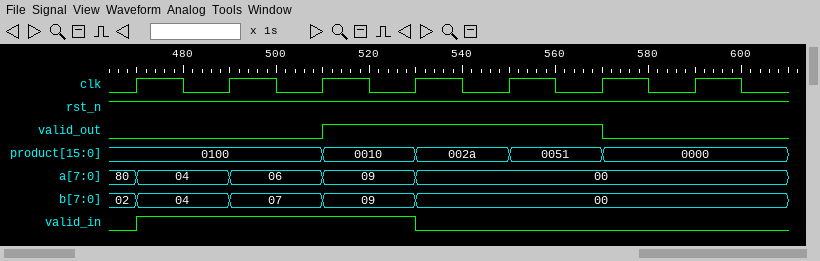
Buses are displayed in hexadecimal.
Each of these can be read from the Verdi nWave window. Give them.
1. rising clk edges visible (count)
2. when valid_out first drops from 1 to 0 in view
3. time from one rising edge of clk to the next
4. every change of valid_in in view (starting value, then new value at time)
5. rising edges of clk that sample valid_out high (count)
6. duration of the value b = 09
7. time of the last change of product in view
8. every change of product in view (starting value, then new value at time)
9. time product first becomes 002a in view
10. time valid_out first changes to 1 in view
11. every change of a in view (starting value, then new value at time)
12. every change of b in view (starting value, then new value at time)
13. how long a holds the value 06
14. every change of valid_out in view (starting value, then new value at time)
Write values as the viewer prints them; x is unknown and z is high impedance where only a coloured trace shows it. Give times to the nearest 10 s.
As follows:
7
570 s
20 s
0, 1 at 470 s, 0 at 530 s
3
20 s
570 s
0100, 0010 at 510 s, 002a at 530 s, 0051 at 550 s, 0000 at 570 s
530 s
510 s
80, 04 at 470 s, 06 at 490 s, 09 at 510 s, 00 at 530 s
02, 04 at 470 s, 07 at 490 s, 09 at 510 s, 00 at 530 s
20 s
0, 1 at 510 s, 0 at 570 s
